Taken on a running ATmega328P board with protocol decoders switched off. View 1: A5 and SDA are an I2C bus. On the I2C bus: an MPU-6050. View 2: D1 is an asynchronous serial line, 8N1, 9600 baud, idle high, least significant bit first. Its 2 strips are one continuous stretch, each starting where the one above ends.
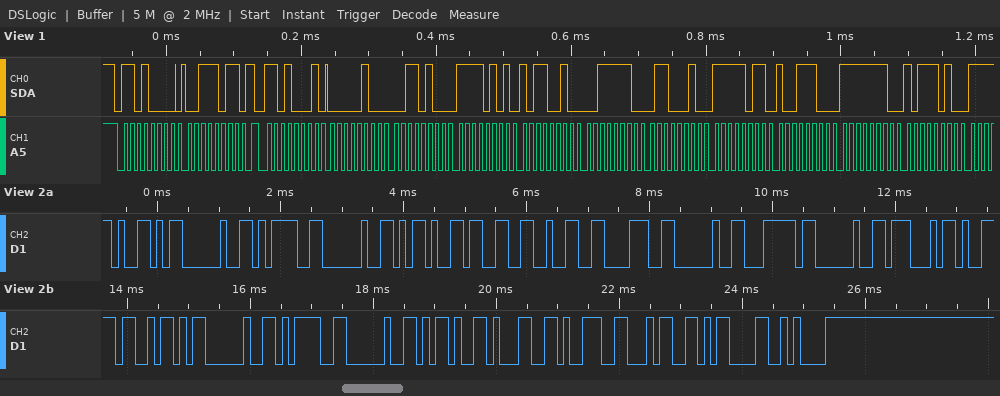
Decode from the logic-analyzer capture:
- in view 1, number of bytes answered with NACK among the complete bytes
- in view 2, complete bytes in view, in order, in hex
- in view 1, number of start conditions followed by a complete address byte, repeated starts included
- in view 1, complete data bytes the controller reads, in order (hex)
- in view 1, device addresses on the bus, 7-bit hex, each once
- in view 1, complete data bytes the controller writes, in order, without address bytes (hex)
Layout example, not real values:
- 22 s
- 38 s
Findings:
- 0
- 0x59 0x20 0x3D 0x20 0x2D 0x33 0x32 0x38 0x20 0x7C 0x20 0x47 0x79 0x5A 0x20 0x3D 0x20 0x2D 0x31 0x39 0x34 0x0D 0x0A
- 2
- 04 34 F5 B2 3E 62 FB 9C FE BA
- 0x68
- 3B
